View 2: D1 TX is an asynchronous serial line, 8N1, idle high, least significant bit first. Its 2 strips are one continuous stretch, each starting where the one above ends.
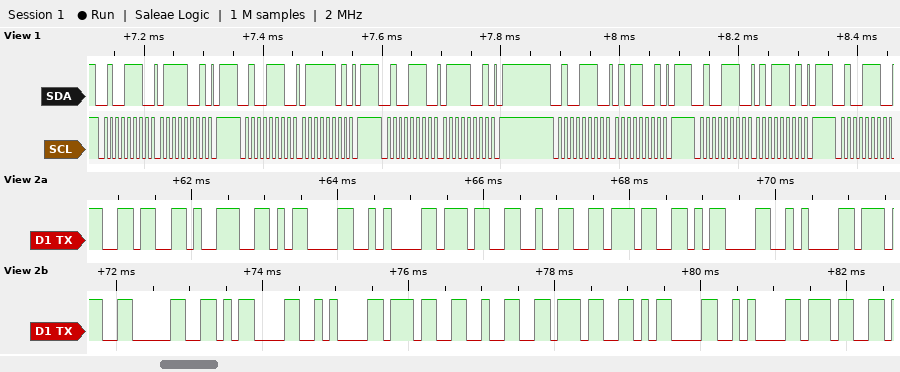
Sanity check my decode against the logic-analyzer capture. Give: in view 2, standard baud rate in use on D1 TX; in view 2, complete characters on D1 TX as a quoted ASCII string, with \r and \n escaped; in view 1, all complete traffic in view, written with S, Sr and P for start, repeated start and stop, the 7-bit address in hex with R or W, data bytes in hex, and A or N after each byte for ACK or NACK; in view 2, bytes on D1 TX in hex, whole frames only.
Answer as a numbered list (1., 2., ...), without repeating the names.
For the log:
1. 9600 baud
2. "69\r\n727\r\n70\r\n727\r\n7"
3. S 27W A 79 A P S 27W A 7D A P S 27W A 79 A P S 27W A 59 A P S 27W A 5D A P S 27W A
4. 36 39 0D 0A 37 32 37 0D 0A 37 30 0D 0A 37 32 37 0D 0A 37
